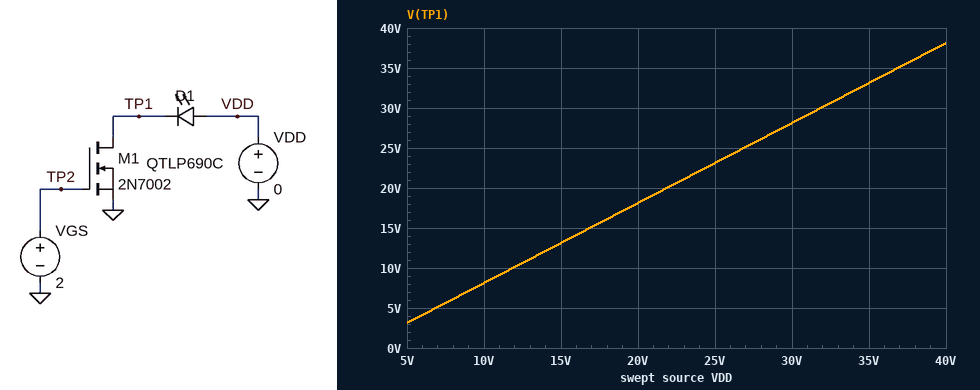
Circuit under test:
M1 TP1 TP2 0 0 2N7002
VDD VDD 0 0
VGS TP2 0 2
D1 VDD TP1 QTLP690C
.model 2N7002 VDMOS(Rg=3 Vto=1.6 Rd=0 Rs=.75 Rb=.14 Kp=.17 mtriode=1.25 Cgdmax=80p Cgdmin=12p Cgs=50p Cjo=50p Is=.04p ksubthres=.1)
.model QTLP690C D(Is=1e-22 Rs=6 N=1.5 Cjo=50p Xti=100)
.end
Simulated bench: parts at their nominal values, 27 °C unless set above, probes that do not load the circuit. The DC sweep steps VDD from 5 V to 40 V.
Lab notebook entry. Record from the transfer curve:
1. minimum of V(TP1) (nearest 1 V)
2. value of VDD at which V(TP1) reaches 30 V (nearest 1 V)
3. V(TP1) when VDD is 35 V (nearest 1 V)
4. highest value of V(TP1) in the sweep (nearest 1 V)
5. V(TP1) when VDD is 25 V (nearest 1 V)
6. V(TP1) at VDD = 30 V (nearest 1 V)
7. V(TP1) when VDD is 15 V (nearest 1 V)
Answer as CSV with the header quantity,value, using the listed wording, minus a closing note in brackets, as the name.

quantity,value
minimum of V(TP1),3 V
value of VDD at which V(TP1) reaches 30 V,32 V
V(TP1) when VDD is 35 V,33 V
highest value of V(TP1) in the sweep,38 V
V(TP1) when VDD is 25 V,23 V
V(TP1) at VDD = 30 V,28 V
V(TP1) when VDD is 15 V,13 V
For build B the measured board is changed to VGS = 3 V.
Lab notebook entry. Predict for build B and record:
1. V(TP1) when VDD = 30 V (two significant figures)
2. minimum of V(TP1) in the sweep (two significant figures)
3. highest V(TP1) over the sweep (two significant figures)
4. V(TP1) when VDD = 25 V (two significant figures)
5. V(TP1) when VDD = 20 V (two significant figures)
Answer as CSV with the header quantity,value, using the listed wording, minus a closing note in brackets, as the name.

quantity,value
V(TP1) when VDD = 30 V,27 V
minimum of V(TP1) in the sweep,2.3 V
highest V(TP1) over the sweep,37 V
V(TP1) when VDD = 25 V,22 V
V(TP1) when VDD = 20 V,17 V
